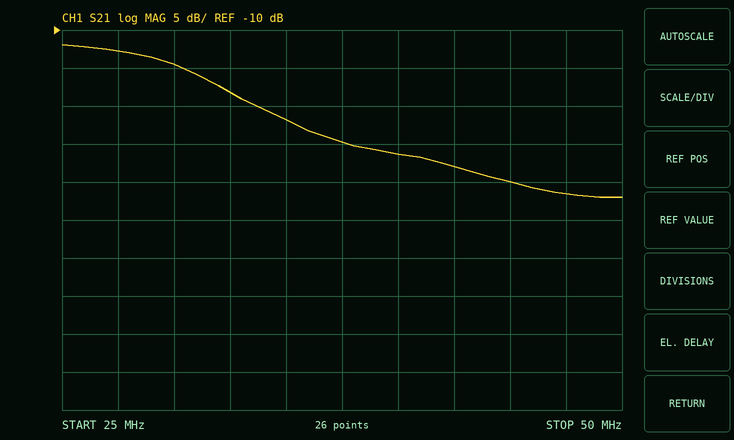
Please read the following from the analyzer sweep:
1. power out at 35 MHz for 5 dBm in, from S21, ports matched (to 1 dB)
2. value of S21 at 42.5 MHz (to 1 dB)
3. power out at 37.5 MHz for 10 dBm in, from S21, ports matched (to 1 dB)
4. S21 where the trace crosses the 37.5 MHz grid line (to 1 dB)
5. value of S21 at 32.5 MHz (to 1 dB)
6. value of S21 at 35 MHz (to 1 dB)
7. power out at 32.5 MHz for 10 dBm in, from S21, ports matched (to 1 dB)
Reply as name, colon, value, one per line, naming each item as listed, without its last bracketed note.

power out at 35 MHz for 5 dBm in, from S21, ports matched: -17 dBm
value of S21 at 42.5 MHz: -28 dB
power out at 37.5 MHz for 10 dBm in, from S21, ports matched: -15 dBm
S21 where the trace crosses the 37.5 MHz grid line: -25 dB
value of S21 at 32.5 MHz: -18 dB
value of S21 at 35 MHz: -22 dB
power out at 32.5 MHz for 10 dBm in, from S21, ports matched: -8 dBm
